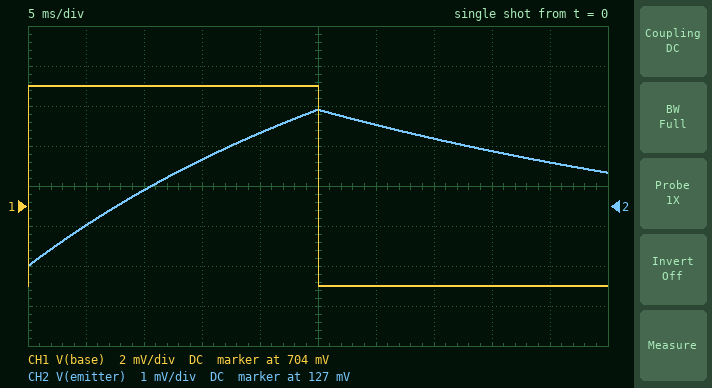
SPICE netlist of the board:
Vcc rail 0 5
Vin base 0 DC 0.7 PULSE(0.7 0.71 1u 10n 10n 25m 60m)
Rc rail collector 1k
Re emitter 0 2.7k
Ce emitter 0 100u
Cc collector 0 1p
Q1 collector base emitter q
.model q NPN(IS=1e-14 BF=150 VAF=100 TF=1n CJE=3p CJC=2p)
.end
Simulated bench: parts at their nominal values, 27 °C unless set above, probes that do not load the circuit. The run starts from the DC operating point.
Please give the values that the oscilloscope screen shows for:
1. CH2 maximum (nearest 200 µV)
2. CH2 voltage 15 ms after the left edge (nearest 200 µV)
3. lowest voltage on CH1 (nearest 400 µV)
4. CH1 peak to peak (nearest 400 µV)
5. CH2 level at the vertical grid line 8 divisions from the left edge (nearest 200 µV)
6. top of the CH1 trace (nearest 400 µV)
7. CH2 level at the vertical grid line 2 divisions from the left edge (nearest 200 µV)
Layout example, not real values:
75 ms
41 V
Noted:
129.4 mV
128.2 mV
700.0 mV
10.0 mV
128.4 mV
710.0 mV
127.4 mV
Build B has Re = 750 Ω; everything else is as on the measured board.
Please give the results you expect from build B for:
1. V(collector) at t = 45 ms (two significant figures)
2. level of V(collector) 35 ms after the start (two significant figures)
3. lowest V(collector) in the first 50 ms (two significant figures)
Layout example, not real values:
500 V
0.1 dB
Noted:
4.9 V
4.9 V
4.8 V
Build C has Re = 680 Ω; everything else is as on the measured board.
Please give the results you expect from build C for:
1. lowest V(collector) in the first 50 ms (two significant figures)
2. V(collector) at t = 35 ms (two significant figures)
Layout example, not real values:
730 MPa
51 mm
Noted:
4.8 V
4.9 V
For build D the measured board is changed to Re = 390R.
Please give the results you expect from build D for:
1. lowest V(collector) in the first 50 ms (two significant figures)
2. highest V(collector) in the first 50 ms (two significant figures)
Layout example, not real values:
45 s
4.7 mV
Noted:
4.7 V
4.8 V
